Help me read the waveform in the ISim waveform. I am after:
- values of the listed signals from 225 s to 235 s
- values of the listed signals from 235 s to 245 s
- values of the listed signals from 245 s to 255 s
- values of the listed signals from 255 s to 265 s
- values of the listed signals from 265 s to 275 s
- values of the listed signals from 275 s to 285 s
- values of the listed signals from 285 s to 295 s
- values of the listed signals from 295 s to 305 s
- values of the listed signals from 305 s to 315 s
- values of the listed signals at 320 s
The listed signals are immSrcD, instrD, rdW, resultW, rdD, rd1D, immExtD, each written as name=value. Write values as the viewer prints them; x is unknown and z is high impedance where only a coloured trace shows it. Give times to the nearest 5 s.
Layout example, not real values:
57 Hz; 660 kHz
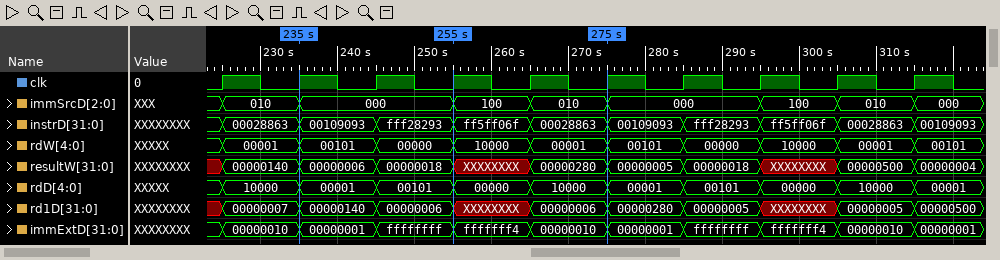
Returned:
immSrcD=010, instrD=00028863, rdW=00001, resultW=00000140, rdD=10000, rd1D=00000007, immExtD=00000010; immSrcD=000, instrD=00109093, rdW=00101, resultW=00000006, rdD=00001, rd1D=00000140, immExtD=00000001; immSrcD=000, instrD=fff28293, rdW=00000, resultW=00000018, rdD=00101, rd1D=00000006, immExtD=ffffffff; immSrcD=100, instrD=ff5ff06f, rdW=10000, resultW=XXXXXXXX, rdD=00000, rd1D=XXXXXXXX, immExtD=fffffff4; immSrcD=010, instrD=00028863, rdW=00001, resultW=00000280, rdD=10000, rd1D=00000006, immExtD=00000010; immSrcD=000, instrD=00109093, rdW=00101, resultW=00000005, rdD=00001, rd1D=00000280, immExtD=00000001; immSrcD=000, instrD=fff28293, rdW=00000, resultW=00000018, rdD=00101, rd1D=00000005, immExtD=ffffffff; immSrcD=100, instrD=ff5ff06f, rdW=10000, resultW=XXXXXXXX, rdD=00000, rd1D=XXXXXXXX, immExtD=fffffff4; immSrcD=010, instrD=00028863, rdW=00001, resultW=00000500, rdD=10000, rd1D=00000005, immExtD=00000010; immSrcD=000, instrD=00109093, rdW=00101, resultW=00000004, rdD=00001, rd1D=00000500, immExtD=00000001
